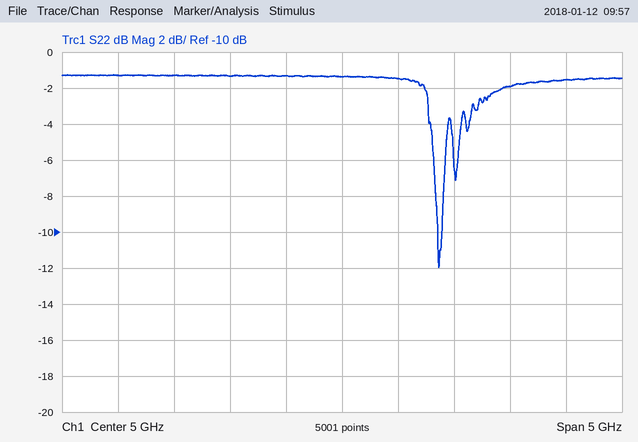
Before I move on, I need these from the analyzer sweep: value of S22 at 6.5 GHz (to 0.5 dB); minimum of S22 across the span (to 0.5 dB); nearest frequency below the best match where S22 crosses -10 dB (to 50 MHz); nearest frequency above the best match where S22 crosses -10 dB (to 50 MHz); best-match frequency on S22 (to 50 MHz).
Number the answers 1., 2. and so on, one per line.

1. -2.0 dB
2. -12.0 dB
3. 5.85 GHz
4. 5.90 GHz
5. 5.85 GHz
